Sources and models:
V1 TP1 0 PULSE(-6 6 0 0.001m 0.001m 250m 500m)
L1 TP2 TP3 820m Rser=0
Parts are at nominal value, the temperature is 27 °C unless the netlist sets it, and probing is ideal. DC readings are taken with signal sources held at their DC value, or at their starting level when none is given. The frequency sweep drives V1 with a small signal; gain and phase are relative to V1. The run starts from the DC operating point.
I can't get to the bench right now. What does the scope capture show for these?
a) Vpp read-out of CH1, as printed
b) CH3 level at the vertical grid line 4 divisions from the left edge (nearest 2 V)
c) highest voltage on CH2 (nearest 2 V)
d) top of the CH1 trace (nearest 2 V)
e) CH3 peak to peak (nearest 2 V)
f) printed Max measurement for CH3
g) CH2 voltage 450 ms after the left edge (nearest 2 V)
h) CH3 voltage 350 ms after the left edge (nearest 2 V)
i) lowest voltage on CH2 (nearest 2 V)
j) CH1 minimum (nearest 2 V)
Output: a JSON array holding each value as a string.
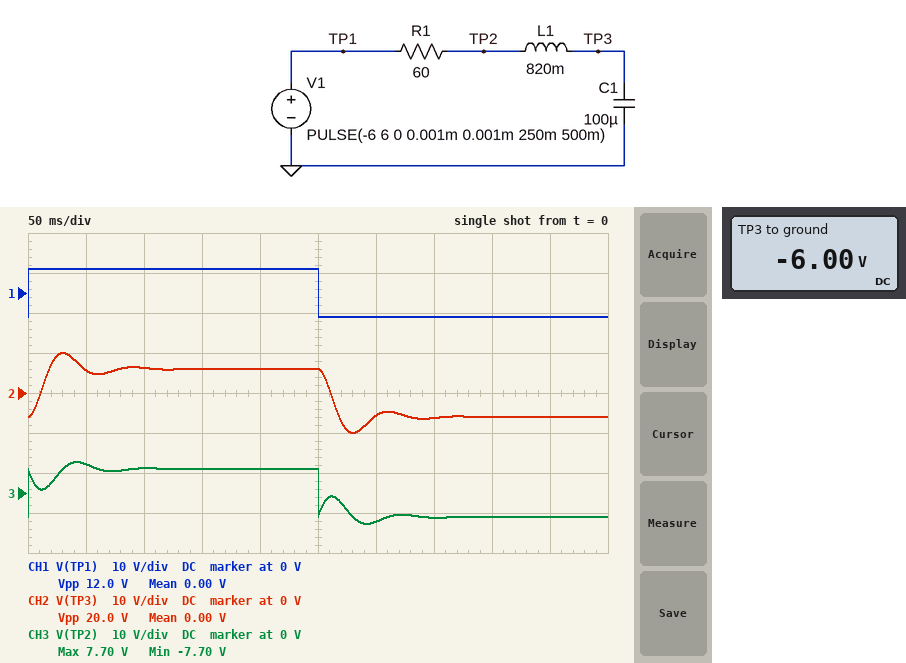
["12.0 V", "6 V", "10 V", "6 V", "16 V", "7.70 V", "-6 V", "-6 V", "-10 V", "-6 V"]
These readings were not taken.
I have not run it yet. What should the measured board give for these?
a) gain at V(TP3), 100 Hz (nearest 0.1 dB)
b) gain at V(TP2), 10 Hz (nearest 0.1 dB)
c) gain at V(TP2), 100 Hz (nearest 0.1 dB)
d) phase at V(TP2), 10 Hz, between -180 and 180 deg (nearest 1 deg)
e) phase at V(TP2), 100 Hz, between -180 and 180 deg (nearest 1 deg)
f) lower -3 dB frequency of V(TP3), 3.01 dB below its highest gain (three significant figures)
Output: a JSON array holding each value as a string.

["-30.0 dB", "-1.2 dB", "-0.1 dB", "-29 deg", "7 deg", "6.93 Hz"]
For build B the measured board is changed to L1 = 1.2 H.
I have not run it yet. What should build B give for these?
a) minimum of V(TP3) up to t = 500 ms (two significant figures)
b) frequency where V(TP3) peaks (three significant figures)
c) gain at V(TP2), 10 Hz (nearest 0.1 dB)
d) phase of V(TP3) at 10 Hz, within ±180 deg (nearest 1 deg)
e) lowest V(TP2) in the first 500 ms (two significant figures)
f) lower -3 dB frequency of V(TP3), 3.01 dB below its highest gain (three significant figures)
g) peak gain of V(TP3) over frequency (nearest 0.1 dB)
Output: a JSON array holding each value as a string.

["-11 V", "13.4 Hz", "-1.8 dB", "-36 deg", "-7.9 V", "8.26 Hz", "5.6 dB"]
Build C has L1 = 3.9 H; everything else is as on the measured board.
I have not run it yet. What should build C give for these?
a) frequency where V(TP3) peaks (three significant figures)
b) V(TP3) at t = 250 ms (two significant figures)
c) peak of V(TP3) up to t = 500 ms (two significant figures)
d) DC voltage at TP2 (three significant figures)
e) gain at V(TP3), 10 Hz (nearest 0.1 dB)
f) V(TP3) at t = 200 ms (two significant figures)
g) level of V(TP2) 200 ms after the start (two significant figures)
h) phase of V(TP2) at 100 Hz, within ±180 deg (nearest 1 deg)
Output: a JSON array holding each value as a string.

["7.87 Hz", "4.3 V", "13 V", "-6.00 V", "3.6 dB", "8.4 V", "6.4 V", "1 deg"]
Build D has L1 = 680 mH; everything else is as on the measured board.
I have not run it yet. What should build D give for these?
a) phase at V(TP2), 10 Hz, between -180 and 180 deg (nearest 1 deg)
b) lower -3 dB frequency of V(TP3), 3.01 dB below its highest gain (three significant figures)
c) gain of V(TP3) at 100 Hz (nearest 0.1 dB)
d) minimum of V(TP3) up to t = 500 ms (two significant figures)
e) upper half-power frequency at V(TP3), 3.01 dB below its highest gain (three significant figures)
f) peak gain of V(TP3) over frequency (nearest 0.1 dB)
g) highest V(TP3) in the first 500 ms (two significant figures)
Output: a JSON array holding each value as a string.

["-27 deg", "4.63 Hz", "-28.3 dB", "-9.5 V", "22.9 Hz", "3.4 dB", "9.5 V"]
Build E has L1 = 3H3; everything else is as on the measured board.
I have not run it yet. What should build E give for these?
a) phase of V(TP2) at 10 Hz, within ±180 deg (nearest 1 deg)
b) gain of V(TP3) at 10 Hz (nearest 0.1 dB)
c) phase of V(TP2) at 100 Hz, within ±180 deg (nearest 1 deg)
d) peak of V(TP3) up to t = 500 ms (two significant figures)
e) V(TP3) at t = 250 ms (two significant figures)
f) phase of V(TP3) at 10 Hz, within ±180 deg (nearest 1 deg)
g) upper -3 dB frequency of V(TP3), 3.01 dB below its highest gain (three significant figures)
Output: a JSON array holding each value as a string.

["51 deg", "6.3 dB", "2 deg", "13 V", "5.2 V", "-129 deg", "9.88 Hz"]
